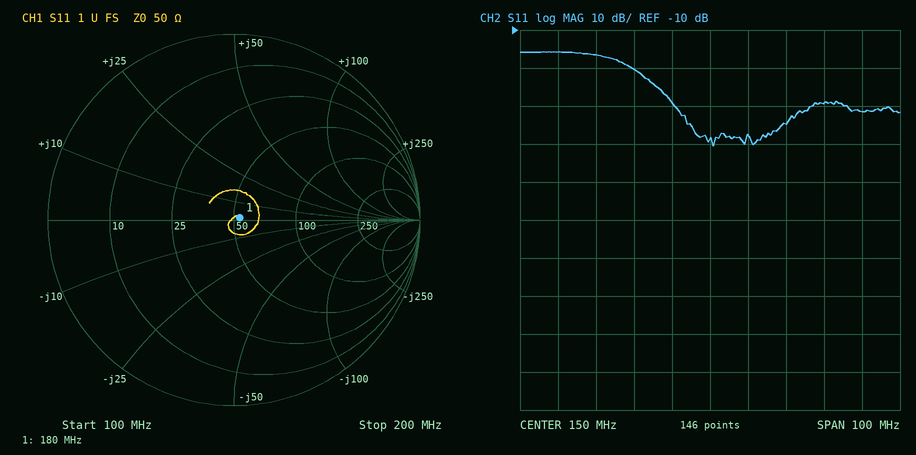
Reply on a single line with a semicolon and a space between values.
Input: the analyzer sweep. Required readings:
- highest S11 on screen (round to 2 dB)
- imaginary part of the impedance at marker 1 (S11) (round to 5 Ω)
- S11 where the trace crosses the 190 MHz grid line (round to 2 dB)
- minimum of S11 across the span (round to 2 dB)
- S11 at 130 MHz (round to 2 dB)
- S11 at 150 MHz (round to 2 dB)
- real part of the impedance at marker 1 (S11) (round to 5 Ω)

-16 dB; 0 Ω; -32 dB; -40 dB; -20 dB; -38 dB; 55 Ω
